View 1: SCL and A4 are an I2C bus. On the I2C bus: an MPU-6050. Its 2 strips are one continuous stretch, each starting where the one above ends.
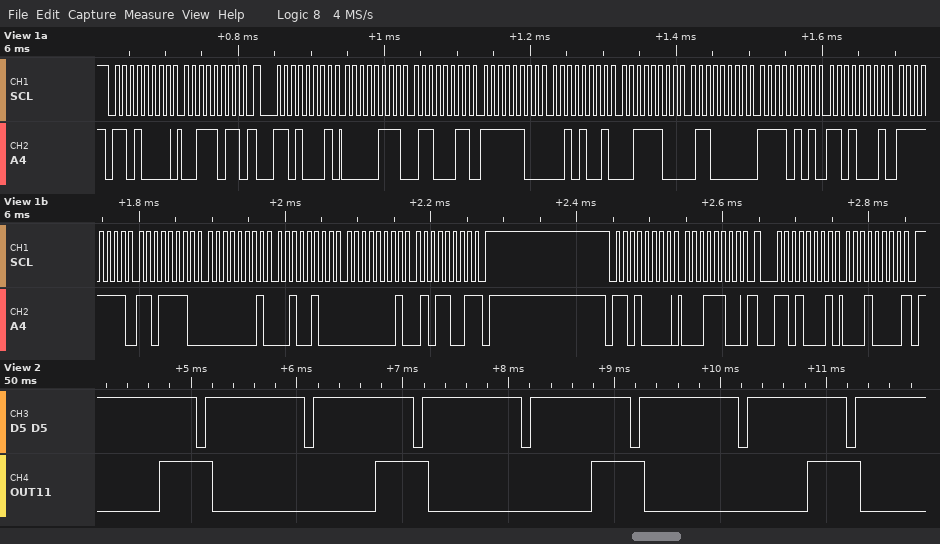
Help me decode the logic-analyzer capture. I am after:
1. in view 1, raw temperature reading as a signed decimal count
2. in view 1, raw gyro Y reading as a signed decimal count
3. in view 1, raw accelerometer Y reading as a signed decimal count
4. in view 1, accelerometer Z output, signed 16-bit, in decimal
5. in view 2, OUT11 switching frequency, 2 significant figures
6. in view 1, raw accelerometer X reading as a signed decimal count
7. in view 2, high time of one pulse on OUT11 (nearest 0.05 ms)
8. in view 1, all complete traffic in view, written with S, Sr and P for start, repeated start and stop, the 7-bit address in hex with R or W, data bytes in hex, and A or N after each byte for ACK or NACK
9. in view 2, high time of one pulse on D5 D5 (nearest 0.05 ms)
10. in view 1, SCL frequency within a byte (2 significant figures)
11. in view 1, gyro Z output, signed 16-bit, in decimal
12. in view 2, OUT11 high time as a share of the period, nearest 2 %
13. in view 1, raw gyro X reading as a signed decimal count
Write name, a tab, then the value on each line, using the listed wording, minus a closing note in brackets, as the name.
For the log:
in view 1, raw temperature reading as a signed decimal count	-2607
in view 1, raw gyro Y reading as a signed decimal count	292
in view 1, raw accelerometer Y reading as a signed decimal count	-983
in view 1, accelerometer Z output, signed 16-bit, in decimal	15456
in view 2, OUT11 switching frequency, 2 significant figures	490 Hz
in view 1, raw accelerometer X reading as a signed decimal count	1891
in view 2, high time of one pulse on OUT11	0.50 ms
in view 1, all complete traffic in view, written with S, Sr and P for start, repeated start and stop, the 7-bit address in hex with R or W, data bytes in hex, and A or N after each byte for ACK or NACK	S 68W A 3B A Sr 68R A 07 A 63 A FC A 29 A 3C A 60 A F5 A D1 A FF A DE A 01 A 24 A 01 A 59 N P S 68W A 1C A Sr 68R A 10 N P
in view 2, high time of one pulse on D5 D5	0.95 ms
in view 1, SCL frequency within a byte	100 kHz
in view 1, gyro Z output, signed 16-bit, in decimal	345
in view 2, OUT11 high time as a share of the period, nearest 2 %	24 %
in view 1, raw gyro X reading as a signed decimal count	-34
